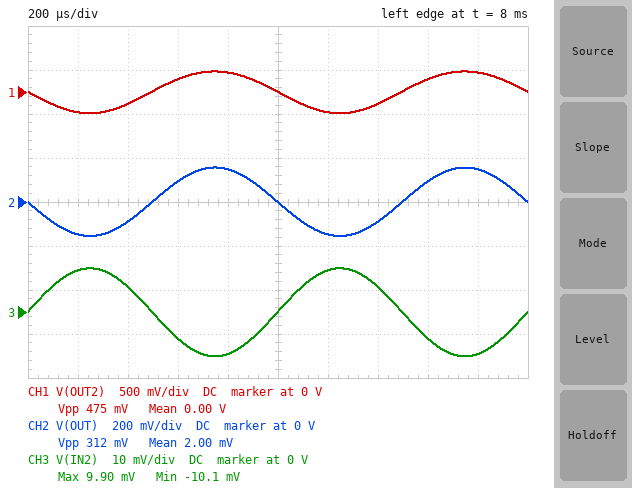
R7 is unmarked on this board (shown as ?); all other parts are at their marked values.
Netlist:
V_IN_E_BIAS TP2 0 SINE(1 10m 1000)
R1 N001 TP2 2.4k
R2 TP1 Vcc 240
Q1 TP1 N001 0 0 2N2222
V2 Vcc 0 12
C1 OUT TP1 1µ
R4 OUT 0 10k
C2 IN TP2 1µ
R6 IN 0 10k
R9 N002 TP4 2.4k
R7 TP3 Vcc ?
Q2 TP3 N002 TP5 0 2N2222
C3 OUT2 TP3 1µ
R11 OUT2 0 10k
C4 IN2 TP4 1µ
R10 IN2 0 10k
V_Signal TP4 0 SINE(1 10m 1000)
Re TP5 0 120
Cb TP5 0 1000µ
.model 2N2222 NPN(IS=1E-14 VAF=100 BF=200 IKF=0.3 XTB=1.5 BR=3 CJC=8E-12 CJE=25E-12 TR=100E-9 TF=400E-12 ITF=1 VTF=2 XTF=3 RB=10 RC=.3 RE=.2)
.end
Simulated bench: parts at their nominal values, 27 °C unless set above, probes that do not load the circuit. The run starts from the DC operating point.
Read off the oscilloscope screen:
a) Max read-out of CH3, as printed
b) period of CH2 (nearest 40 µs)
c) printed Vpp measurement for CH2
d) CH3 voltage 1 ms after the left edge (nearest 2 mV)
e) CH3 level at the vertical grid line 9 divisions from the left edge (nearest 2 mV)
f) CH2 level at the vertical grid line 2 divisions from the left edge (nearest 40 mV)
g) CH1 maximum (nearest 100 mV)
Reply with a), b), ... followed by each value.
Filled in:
a) 9.90 mV
b) 1.00 ms
c) 312 mV
d) 0 V
e) -10 mV
f) -80 mV
g) 200 mV
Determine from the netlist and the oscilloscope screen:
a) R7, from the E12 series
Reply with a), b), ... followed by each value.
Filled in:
a) 560 Ω
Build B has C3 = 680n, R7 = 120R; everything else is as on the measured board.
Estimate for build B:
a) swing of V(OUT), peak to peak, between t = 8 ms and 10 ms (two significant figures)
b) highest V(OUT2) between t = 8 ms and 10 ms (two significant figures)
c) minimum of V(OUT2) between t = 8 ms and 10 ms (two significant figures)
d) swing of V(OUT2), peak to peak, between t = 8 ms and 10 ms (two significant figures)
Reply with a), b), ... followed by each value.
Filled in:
a) 310 mV
b) 53 mV
c) -55 mV
d) 110 mV
